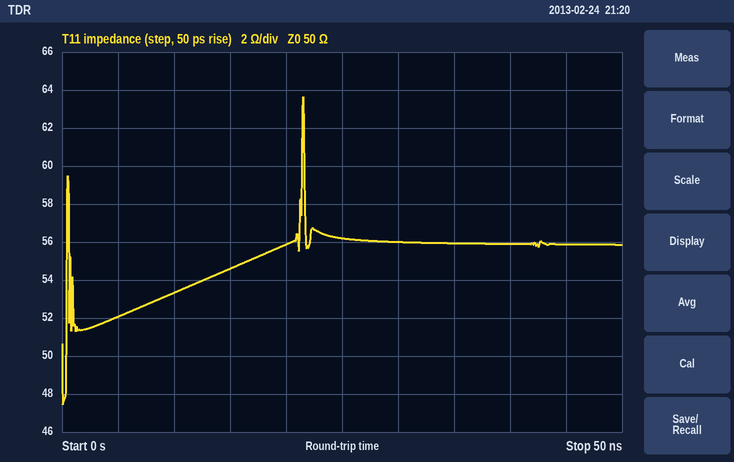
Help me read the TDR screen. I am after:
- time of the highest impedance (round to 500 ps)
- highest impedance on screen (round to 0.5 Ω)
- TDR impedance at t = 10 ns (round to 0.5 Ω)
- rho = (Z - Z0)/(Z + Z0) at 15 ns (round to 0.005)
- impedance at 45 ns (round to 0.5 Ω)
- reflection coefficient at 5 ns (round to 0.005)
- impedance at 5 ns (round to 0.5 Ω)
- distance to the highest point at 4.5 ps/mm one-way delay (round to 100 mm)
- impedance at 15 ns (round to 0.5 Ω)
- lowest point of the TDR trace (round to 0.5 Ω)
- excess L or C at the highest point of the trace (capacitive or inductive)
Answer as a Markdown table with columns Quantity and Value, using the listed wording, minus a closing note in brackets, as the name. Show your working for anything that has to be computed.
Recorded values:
| Quantity | Value |
|---|---|
| time of the highest impedance | 21.5 ns |
| highest impedance on screen | 63.5 Ω |
| TDR impedance at t = 10 ns | 53.5 Ω |
| rho = (Z - Z0)/(Z + Z0) at 15 ns | (54.5 − 50)/(54.5 + 50) ≈ +0.0431, so +0.045 to the nearest 0.005 |
| impedance at 45 ns | 56.0 Ω |
| reflection coefficient at 5 ns | (52 − 50)/(52 + 50) ≈ +0.020 |
| impedance at 5 ns | 52.0 Ω |
| distance to the highest point at 4.5 ps/mm one-way delay | 21.5 ns / 2 / 4.5 ps/mm ≈ 2.4 m |
| impedance at 15 ns | 54.5 Ω |
| lowest point of the TDR trace | 47.5 Ω |
| excess L or C at the highest point of the trace | inductive |
